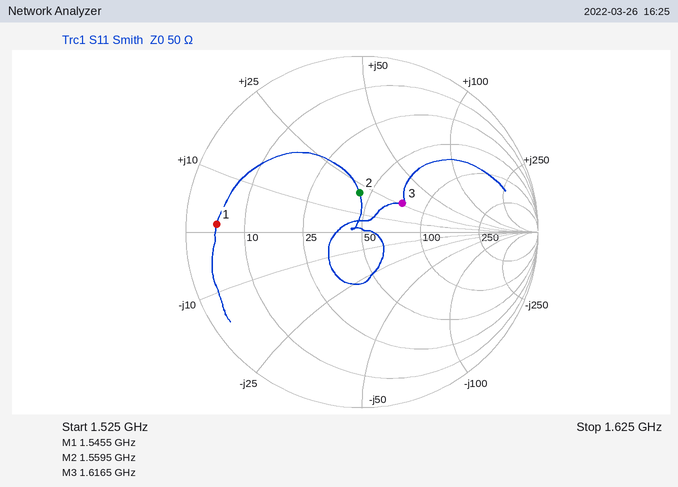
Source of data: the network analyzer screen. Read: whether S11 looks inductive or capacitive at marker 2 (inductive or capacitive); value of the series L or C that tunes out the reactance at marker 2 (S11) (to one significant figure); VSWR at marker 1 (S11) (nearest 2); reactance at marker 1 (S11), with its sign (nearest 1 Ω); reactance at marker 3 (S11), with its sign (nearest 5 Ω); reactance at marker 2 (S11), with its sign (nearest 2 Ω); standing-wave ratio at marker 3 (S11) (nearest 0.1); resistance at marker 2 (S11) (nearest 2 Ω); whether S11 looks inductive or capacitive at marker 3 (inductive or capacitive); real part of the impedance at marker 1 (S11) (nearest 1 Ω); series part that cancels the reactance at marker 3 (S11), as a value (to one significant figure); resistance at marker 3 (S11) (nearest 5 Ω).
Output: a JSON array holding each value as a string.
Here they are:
["inductive", "5 pF", "10", "+1 Ω", "+25 Ω", "+20 Ω", "1.8", "44 Ω", "inductive", "5 Ω", "4 pF", "75 Ω"]
